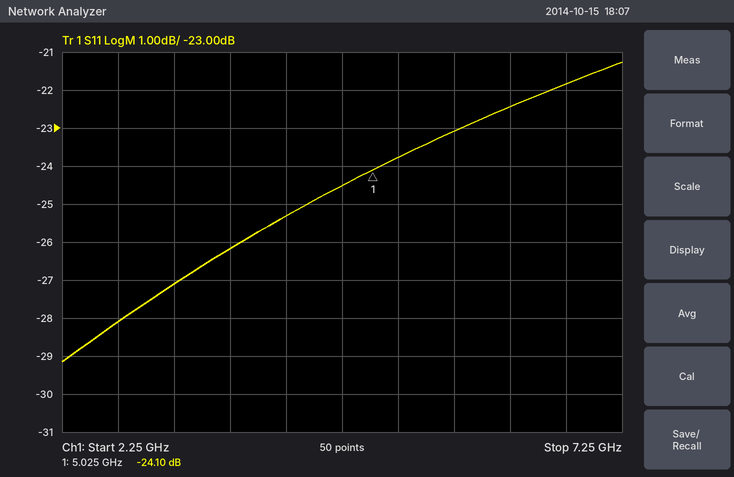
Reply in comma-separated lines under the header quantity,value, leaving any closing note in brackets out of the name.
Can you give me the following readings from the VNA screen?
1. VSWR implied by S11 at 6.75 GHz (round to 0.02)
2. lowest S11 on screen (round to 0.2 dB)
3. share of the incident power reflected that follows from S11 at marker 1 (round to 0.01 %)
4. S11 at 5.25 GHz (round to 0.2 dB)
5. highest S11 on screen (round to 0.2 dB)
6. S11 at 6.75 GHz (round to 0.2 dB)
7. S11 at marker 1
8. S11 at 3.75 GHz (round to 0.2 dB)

quantity,value
VSWR implied by S11 at 6.75 GHz,1.18
lowest S11 on screen,-29.2 dB
share of the incident power reflected that follows from S11 at marker 1,0.39 %
S11 at 5.25 GHz,-23.8 dB
highest S11 on screen,-21.2 dB
S11 at 6.75 GHz,-21.8 dB
S11 at marker 1,-24.10 dB
S11 at 3.75 GHz,-26.2 dB
